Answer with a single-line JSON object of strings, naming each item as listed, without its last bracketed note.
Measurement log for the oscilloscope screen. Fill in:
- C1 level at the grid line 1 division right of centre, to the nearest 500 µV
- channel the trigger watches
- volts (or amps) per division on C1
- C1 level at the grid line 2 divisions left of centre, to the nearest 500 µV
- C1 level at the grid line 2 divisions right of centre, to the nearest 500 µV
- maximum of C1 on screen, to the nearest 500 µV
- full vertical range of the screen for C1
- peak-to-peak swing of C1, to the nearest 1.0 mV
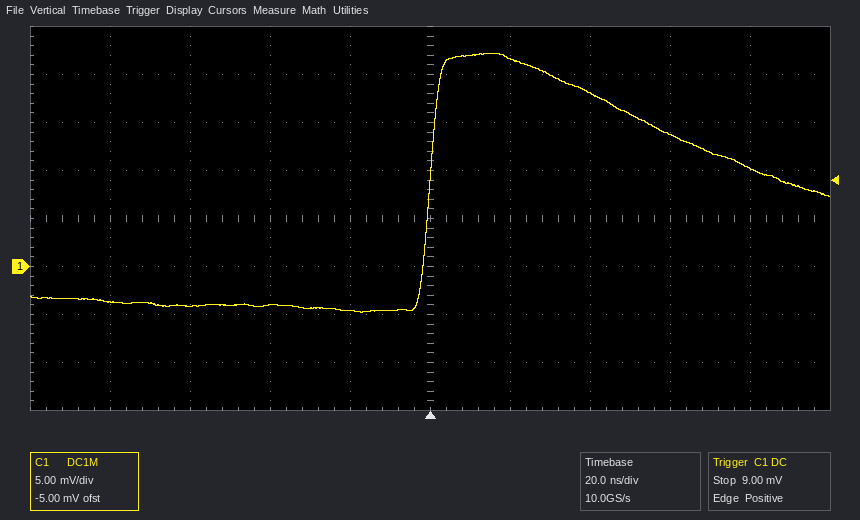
{"C1 level at the grid line 1 division right of centre, to the nearest 500 µV": "21.5 mV", "channel the trigger watches": "C1", "volts (or amps) per division on C1": "5 mV", "C1 level at the grid line 2 divisions left of centre, to the nearest 500 µV": "-4.0 mV", "C1 level at the grid line 2 divisions right of centre, to the nearest 500 µV": "18.0 mV", "maximum of C1 on screen, to the nearest 500 µV": "22.0 mV", "full vertical range of the screen for C1": "40 mV", "peak-to-peak swing of C1, to the nearest 1.0 mV": "27.0 mV"}
